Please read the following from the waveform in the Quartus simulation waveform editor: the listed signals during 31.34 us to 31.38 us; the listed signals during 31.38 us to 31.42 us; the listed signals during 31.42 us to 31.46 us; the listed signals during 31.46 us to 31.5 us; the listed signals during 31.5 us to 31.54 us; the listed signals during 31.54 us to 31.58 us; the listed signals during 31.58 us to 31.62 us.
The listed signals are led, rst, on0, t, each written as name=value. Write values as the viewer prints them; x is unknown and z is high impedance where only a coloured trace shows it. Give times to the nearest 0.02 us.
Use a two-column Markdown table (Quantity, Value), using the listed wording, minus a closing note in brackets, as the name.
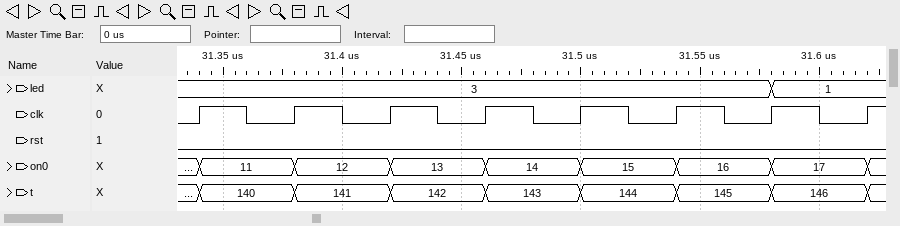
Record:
| Quantity | Value |
|---|---|
| the listed signals during 31.34 us to 31.38 us | led=3, rst=0, on0=11, t=140 |
| the listed signals during 31.38 us to 31.42 us | led=3, rst=0, on0=12, t=141 |
| the listed signals during 31.42 us to 31.46 us | led=3, rst=0, on0=13, t=142 |
| the listed signals during 31.46 us to 31.5 us | led=3, rst=0, on0=14, t=143 |
| the listed signals during 31.5 us to 31.54 us | led=3, rst=0, on0=15, t=144 |
| the listed signals during 31.54 us to 31.58 us | led=3, rst=0, on0=16, t=145 |
| the listed signals during 31.58 us to 31.62 us | led=1, rst=0, on0=17, t=146 |
